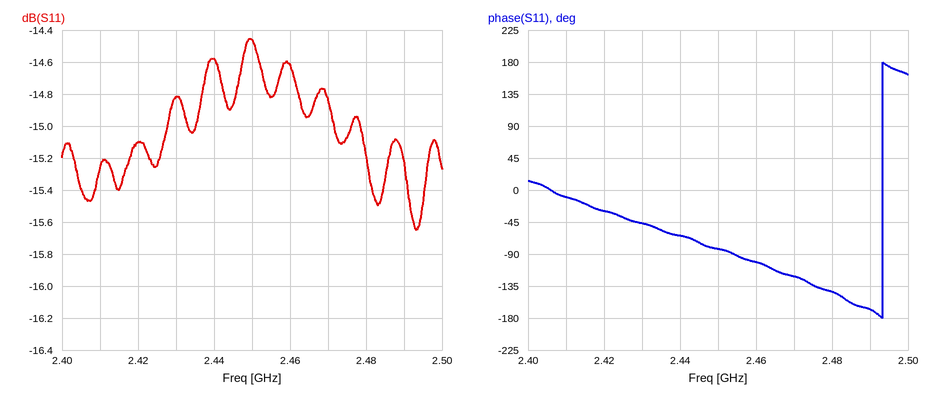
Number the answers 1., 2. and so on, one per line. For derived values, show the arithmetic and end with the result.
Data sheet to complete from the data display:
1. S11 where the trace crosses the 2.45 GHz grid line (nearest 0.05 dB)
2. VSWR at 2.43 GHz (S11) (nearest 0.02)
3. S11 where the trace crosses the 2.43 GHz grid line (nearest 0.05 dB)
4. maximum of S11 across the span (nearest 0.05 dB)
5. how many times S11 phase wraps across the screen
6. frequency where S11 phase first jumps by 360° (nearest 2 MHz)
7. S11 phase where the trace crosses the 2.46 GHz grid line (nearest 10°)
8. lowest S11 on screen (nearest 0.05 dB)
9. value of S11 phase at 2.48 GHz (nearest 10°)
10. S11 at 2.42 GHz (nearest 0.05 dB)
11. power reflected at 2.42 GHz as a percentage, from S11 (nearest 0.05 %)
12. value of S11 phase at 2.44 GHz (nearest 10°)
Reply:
1. -14.45 dB
2. |Γ| = 10^(-14.8/20) = 0.1820; VSWR = (1 + 0.1820)/(1 − 0.1820) ≈ 1.44
3. -14.80 dB
4. -14.45 dB
5. 1
6. 2.494 GHz
7. -100°
8. -15.65 dB
9. -140°
10. -15.10 dB
11. 10^(-15.1/10) ≈ 3.09 %, so 3.10 % to the nearest 0.05 %
12. -60°
